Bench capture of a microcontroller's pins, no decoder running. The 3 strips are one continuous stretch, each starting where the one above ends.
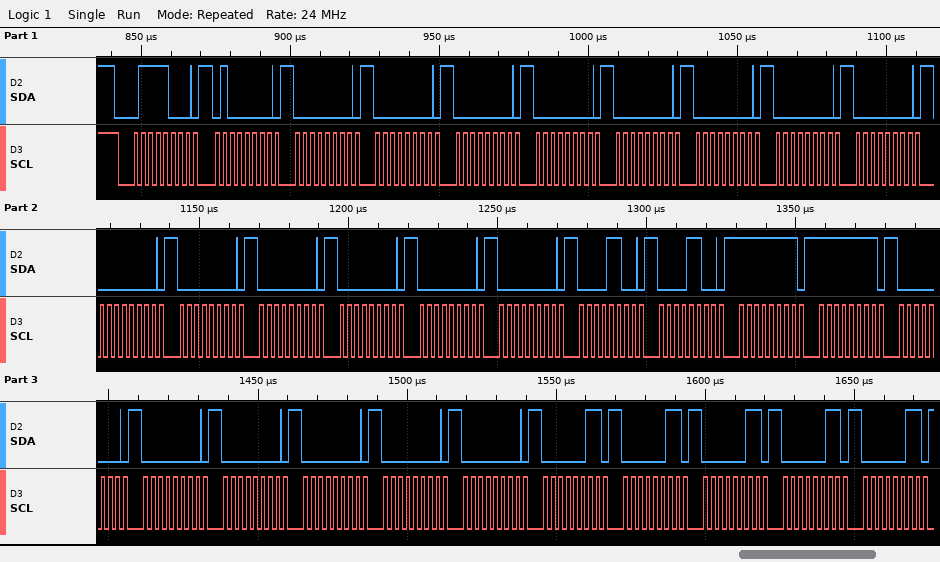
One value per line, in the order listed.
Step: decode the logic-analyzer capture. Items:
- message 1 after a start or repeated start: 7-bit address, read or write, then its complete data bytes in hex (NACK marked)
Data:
0x3C write: 40 00 00 00 00 00 00 00 00 00 00 00 00 00 00 0C 0C FF FF 00 00 00 00 00 00 03 03 03 03 03
